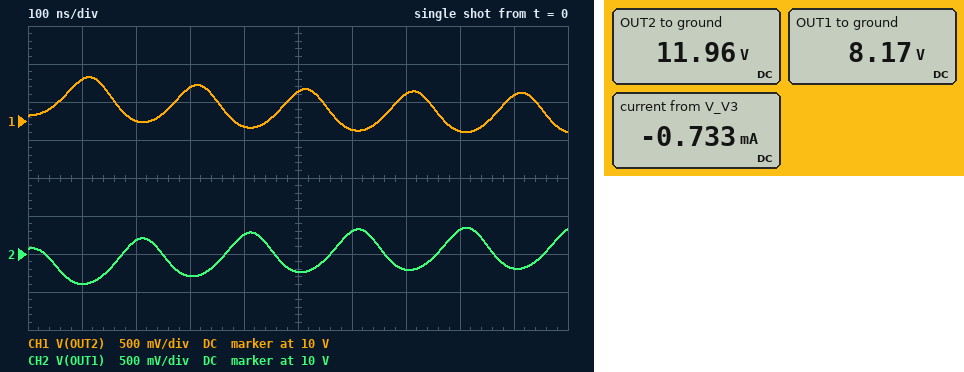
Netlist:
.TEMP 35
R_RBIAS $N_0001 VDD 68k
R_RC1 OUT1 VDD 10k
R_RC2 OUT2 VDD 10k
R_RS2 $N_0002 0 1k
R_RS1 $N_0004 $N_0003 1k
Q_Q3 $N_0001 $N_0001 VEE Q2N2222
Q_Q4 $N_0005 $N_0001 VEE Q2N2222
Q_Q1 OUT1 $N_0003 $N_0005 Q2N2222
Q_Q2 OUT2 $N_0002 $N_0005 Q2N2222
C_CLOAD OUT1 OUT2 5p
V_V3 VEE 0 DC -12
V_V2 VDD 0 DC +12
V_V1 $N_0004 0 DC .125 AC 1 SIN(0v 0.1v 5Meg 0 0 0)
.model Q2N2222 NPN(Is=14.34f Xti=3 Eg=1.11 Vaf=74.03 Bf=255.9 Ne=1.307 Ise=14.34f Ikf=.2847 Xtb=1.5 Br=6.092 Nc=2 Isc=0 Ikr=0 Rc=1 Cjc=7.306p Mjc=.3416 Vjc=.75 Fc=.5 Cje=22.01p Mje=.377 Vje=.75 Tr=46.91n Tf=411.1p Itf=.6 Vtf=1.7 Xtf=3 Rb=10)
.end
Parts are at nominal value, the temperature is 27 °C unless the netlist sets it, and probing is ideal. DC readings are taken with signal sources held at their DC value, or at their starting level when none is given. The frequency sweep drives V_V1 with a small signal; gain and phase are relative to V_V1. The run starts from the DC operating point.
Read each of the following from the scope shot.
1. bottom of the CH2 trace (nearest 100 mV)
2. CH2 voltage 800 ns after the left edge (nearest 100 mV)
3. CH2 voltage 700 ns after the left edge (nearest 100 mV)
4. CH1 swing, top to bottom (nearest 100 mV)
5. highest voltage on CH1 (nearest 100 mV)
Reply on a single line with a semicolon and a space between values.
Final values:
9.6 V; 10.3 V; 9.8 V; 700 mV; 10.6 V
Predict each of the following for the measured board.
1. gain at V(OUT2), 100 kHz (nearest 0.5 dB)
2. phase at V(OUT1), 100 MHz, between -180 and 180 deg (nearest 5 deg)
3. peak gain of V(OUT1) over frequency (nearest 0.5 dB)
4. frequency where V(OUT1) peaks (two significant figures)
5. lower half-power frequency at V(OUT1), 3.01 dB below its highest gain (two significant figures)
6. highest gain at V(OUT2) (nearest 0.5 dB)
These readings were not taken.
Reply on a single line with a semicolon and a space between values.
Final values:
3.5 dB; -15 deg; 9.5 dB; 4.1 MHz; 1.4 MHz; 5.5 dB
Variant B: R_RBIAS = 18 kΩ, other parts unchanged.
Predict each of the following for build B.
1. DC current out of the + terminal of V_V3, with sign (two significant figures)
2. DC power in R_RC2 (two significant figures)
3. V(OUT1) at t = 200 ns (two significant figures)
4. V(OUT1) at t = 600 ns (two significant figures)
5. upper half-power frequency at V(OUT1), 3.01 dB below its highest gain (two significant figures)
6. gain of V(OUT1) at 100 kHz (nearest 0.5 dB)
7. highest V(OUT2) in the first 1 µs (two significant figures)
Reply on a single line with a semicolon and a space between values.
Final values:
-2.8 mA; 240 µW; 4.8 V; 4.9 V; 23 MHz; -15.0 dB; 5.4 V
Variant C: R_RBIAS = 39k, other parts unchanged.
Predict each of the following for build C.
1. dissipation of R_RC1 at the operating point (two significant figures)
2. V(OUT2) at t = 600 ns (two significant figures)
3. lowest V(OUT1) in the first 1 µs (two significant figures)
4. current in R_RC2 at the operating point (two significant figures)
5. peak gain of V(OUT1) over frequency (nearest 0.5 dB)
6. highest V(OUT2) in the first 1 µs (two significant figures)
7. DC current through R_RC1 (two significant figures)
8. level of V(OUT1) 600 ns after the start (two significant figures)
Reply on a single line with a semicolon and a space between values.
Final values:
4.4 mW; 8.4 V; 8.0 V; 7.7 µA; 9.5 dB; 9.3 V; 670 µA; 8.9 V
